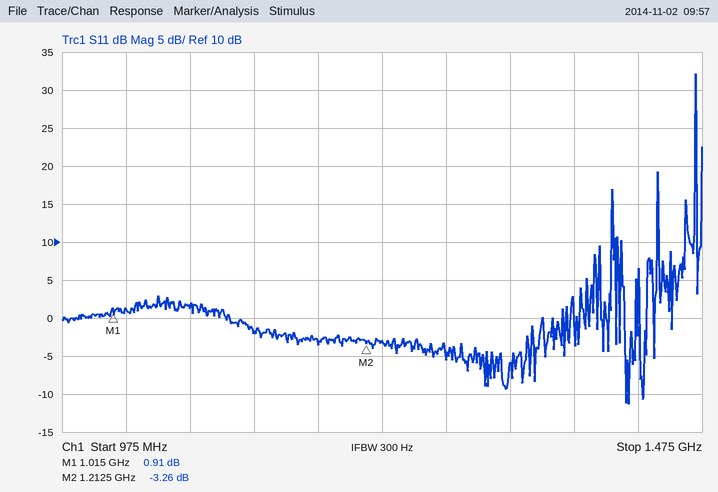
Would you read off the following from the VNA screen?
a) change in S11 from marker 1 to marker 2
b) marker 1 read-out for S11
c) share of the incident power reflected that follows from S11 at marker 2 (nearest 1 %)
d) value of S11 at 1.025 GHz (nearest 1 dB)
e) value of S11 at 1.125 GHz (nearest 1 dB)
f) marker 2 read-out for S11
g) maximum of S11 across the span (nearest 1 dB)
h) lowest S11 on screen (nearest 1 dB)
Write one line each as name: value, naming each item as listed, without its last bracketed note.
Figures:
change in S11 from marker 1 to marker 2: -4.17 dB
marker 1 read-out for S11: 0.91 dB
share of the incident power reflected that follows from S11 at marker 2: 47 %
value of S11 at 1.025 GHz: 1 dB
value of S11 at 1.125 GHz: -2 dB
marker 2 read-out for S11: -3.26 dB
maximum of S11 across the span: 32 dB
lowest S11 on screen: -11 dB
